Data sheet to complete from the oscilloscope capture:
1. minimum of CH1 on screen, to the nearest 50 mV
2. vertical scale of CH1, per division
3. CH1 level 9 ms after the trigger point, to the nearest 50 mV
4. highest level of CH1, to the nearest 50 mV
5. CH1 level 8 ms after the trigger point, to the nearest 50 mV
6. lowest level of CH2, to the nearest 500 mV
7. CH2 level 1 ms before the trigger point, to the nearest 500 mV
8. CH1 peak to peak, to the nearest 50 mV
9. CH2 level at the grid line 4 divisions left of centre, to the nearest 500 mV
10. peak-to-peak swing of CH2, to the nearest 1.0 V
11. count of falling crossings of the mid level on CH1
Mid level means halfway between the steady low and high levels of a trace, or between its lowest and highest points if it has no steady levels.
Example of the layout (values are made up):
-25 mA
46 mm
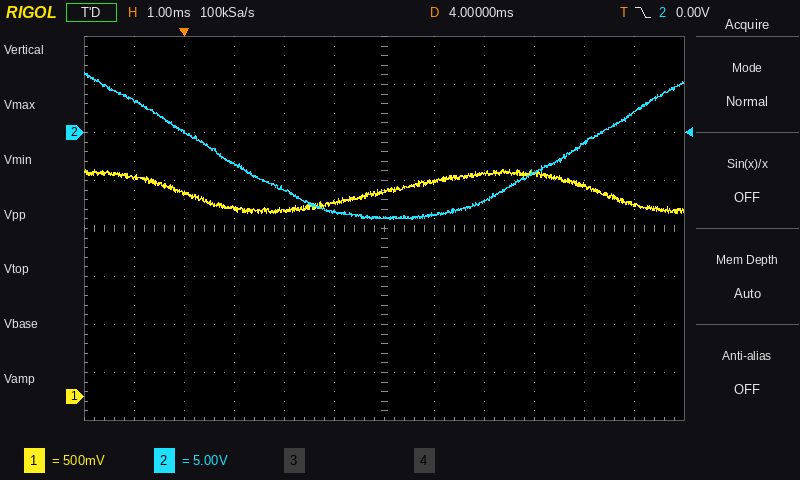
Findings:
1.90 V
500 mV
2.00 V
2.35 V
2.20 V
-9.0 V
3.5 V
450 mV
0.0 V
15.0 V
2
